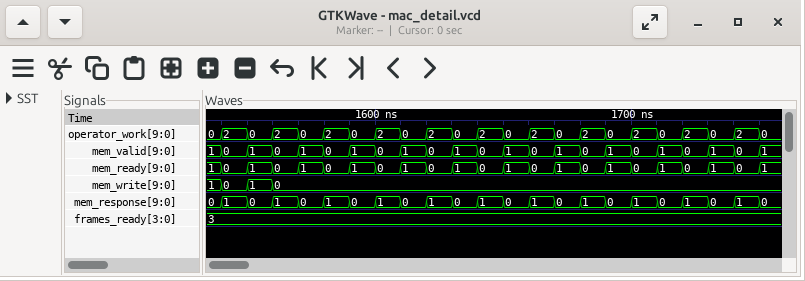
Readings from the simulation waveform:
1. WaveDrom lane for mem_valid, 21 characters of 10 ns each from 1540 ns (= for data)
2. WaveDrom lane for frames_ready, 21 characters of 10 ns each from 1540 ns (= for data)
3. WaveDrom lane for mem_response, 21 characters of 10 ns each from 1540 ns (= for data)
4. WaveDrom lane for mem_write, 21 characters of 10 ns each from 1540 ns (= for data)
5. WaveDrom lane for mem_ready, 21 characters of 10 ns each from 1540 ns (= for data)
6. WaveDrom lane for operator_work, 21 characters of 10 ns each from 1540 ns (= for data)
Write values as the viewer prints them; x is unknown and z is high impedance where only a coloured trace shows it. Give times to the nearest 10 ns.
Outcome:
{name: 'mem_valid', wave: '=====================', data: '0 1 0 1 0 1 0 1 0 1 0 1 0 1 0 1 0 1 0 1 0'}
{name: 'frames_ready', wave: '=....................', data: '3'}
{name: 'mem_response', wave: '=====================', data: '1 0 1 0 1 0 1 0 1 0 1 0 1 0 1 0 1 0 1 0 1'}
{name: 'mem_write', wave: '===..................', data: '0 1 0'}
{name: 'mem_ready', wave: '=====================', data: '0 1 0 1 0 1 0 1 0 1 0 1 0 1 0 1 0 1 0 1 0'}
{name: 'operator_work', wave: '=====================', data: '2 0 2 0 2 0 2 0 2 0 2 0 2 0 2 0 2 0 2 0 2'}
